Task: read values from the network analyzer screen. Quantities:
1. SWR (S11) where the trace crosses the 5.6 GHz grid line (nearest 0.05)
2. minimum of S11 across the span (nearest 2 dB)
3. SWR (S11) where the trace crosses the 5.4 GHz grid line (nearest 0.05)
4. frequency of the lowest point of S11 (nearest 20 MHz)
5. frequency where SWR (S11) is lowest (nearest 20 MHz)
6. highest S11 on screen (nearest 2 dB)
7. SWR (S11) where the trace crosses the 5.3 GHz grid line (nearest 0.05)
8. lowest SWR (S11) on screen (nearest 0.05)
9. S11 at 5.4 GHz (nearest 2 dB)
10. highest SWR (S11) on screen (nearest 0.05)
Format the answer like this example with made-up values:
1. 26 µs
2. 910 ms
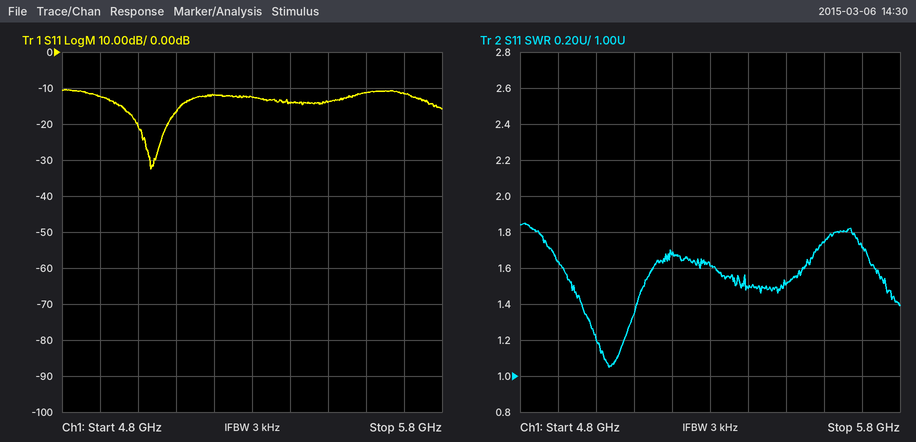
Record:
1. 1.75
2. -32 dB
3. 1.50
4. 5.04 GHz
5. 5.04 GHz
6. -10 dB
7. 1.60
8. 1.05
9. -14 dB
10. 1.85
